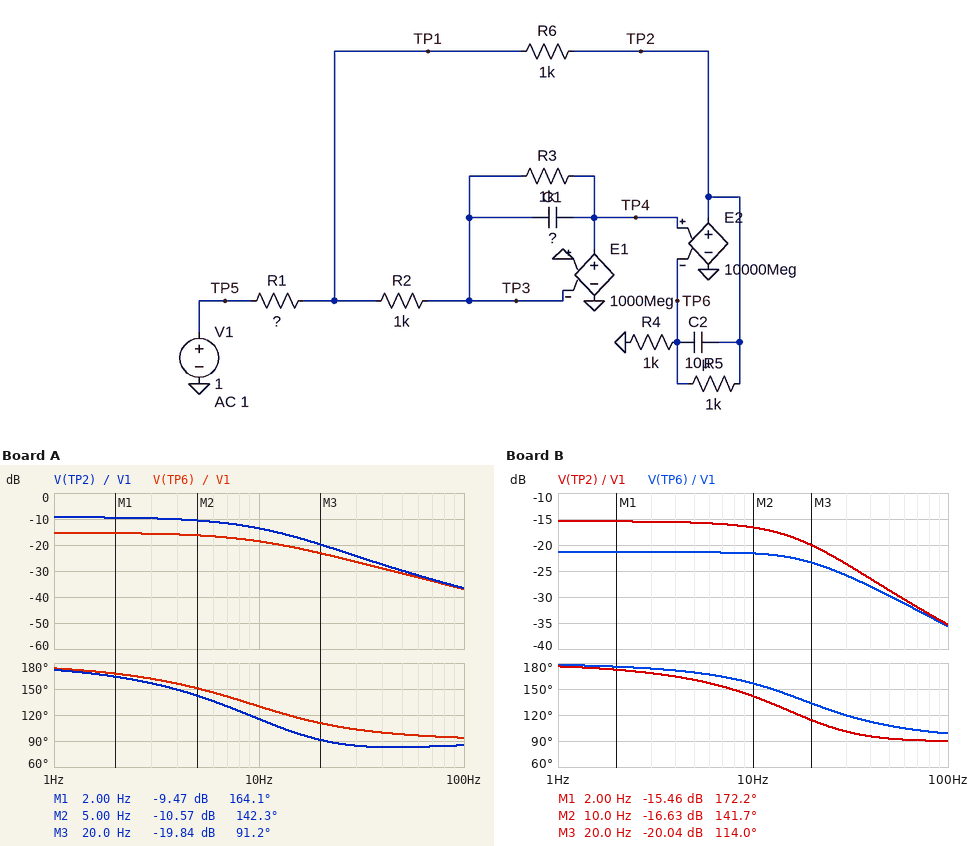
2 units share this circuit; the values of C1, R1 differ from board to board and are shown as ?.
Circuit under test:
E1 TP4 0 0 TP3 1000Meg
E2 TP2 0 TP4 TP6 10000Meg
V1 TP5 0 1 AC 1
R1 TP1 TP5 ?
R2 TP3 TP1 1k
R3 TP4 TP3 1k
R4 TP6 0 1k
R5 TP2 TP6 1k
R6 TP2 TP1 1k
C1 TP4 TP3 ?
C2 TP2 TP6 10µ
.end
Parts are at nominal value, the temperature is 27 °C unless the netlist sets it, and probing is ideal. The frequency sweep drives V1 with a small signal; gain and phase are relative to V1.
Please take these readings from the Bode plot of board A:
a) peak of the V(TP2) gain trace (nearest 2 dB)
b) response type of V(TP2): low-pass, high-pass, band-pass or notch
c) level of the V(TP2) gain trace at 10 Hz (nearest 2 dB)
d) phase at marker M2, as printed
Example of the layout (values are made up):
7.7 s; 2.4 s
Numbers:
-10 dB; low-pass; -14 dB; 142.3 deg
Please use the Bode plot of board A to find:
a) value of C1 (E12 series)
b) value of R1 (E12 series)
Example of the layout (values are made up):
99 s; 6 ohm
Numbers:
33 µF; 1.2 kΩ
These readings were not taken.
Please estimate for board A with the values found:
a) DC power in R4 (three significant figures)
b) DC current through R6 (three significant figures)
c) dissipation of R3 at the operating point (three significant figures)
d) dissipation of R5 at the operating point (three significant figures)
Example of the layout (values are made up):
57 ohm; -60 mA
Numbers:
29.7 µW; 517 µA; 29.7 µW; 29.7 µW
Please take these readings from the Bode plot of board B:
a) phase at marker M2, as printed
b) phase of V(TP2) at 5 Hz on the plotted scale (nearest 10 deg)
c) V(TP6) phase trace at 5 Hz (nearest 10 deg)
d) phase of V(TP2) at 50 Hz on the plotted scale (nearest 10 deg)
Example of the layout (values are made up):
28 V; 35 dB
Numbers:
141.7 deg; 160 deg; 170 deg; 90 deg
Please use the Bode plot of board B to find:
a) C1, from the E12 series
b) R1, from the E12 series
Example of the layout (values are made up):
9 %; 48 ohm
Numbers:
15 µF; 2.7 kΩ
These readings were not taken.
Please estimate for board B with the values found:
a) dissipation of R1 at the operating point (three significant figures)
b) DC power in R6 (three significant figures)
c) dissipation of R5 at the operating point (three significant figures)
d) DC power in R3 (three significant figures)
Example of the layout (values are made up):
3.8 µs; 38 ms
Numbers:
310 µW; 64.6 µW; 7.18 µW; 7.18 µW
